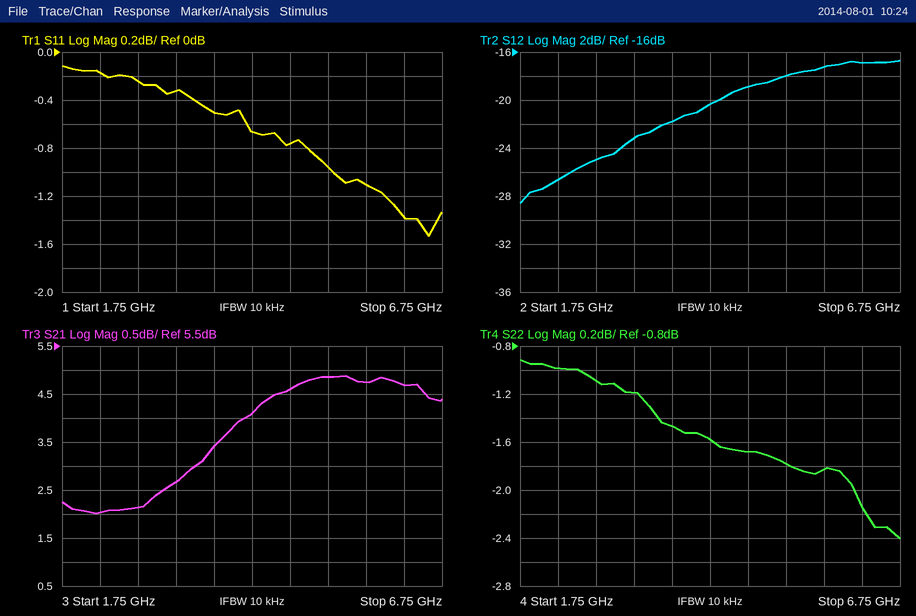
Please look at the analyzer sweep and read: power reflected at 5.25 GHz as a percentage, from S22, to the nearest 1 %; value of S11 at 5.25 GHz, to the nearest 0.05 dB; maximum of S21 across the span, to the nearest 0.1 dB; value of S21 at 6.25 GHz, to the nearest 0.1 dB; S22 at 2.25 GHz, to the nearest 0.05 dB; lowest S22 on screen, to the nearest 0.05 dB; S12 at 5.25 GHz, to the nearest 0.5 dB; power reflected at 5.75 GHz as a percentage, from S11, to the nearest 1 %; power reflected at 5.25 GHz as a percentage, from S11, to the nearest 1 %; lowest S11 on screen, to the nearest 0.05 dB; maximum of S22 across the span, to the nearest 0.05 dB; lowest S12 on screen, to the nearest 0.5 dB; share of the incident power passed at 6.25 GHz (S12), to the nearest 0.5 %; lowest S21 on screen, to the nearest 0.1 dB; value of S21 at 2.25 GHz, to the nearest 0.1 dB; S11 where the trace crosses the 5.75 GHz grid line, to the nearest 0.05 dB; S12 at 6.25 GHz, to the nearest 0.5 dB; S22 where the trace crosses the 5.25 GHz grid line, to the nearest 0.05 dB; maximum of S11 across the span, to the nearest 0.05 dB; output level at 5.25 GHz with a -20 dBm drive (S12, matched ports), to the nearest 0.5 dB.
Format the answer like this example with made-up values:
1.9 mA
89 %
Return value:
66 %
-0.95 dB
4.9 dB
4.7 dB
-1.00 dB
-2.40 dB
-18.0 dB
78 %
80 %
-1.55 dB
-0.90 dB
-28.5 dB
2.0 %
2.0 dB
2.0 dB
-1.10 dB
-17.0 dB
-1.80 dB
-0.10 dB
-38.0 dBm
